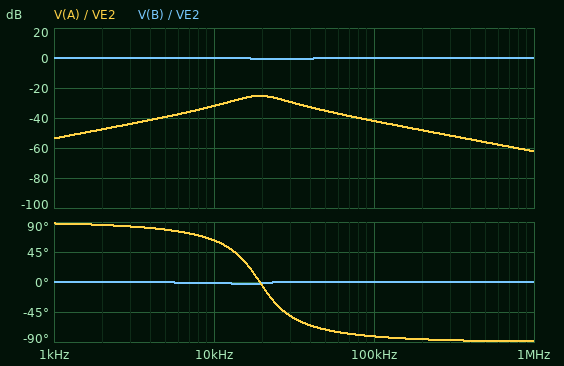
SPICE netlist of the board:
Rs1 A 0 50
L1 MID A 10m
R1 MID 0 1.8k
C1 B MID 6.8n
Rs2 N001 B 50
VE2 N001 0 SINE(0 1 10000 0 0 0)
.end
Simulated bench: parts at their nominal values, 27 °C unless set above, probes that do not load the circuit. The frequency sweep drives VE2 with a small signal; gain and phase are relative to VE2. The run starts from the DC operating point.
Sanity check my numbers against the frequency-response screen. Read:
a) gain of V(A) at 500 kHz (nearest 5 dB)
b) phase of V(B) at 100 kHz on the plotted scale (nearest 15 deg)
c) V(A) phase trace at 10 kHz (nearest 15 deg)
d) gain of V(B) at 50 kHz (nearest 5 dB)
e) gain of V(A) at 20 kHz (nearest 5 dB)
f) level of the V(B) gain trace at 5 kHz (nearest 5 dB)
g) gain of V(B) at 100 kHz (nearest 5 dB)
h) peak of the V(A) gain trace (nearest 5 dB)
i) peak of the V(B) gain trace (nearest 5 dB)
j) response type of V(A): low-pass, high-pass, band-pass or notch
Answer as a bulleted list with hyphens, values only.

- -55 dB
- 0 deg
- 60 deg
- 0 dB
- -25 dB
- 0 dB
- 0 dB
- -25 dB
- 0 dB
- band-pass
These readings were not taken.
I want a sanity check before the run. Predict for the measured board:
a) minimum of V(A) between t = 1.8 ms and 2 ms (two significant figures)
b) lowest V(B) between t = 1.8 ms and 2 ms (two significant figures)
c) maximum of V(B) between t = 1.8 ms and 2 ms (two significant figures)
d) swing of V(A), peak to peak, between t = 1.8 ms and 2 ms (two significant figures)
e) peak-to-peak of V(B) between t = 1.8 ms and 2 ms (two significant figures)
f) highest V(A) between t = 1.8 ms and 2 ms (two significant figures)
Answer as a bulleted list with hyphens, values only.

- -25 mV
- -1.0 V
- 1.0 V
- 50 mV
- 2.0 V
- 25 mV
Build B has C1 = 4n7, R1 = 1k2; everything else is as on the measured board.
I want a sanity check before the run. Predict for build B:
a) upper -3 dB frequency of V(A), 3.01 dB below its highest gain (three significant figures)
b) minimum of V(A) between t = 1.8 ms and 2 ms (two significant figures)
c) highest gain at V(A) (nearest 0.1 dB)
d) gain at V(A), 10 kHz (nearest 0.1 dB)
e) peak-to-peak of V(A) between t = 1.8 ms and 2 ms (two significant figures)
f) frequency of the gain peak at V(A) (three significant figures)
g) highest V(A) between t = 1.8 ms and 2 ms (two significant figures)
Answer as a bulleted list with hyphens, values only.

- 41.6 kHz
- -15 mV
- -31.5 dB
- -36.7 dB
- 29 mV
- 23.2 kHz
- 15 mV
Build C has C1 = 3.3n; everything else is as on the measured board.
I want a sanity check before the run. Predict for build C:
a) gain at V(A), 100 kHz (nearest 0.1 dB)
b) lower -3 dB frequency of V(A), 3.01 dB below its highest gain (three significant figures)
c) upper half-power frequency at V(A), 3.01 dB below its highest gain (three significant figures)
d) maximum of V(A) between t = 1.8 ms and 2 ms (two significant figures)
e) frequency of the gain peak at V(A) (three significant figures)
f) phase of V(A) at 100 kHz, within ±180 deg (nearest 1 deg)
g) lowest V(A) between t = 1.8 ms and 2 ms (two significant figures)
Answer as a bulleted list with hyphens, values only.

- -41.9 dB
- 17.1 kHz
- 44.8 kHz
- 11 mV
- 27.7 kHz
- -73 deg
- -11 mV
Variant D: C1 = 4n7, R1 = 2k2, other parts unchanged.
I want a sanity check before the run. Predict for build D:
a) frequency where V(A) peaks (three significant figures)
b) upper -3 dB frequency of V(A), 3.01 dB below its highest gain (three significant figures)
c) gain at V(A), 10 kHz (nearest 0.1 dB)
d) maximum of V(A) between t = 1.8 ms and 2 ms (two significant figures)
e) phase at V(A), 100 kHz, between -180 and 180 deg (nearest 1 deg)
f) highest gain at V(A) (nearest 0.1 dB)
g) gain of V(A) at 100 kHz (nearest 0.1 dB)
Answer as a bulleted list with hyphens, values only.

- 23.2 kHz
- 33.0 kHz
- -35.6 dB
- 17 mV
- -80 deg
- -26.6 dB
- -41.8 dB
